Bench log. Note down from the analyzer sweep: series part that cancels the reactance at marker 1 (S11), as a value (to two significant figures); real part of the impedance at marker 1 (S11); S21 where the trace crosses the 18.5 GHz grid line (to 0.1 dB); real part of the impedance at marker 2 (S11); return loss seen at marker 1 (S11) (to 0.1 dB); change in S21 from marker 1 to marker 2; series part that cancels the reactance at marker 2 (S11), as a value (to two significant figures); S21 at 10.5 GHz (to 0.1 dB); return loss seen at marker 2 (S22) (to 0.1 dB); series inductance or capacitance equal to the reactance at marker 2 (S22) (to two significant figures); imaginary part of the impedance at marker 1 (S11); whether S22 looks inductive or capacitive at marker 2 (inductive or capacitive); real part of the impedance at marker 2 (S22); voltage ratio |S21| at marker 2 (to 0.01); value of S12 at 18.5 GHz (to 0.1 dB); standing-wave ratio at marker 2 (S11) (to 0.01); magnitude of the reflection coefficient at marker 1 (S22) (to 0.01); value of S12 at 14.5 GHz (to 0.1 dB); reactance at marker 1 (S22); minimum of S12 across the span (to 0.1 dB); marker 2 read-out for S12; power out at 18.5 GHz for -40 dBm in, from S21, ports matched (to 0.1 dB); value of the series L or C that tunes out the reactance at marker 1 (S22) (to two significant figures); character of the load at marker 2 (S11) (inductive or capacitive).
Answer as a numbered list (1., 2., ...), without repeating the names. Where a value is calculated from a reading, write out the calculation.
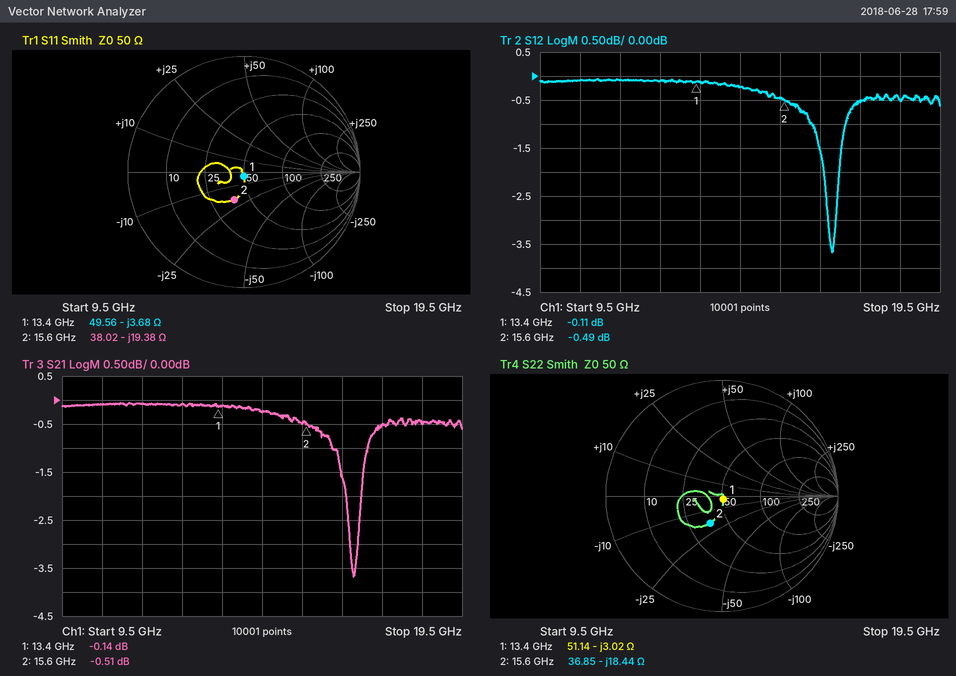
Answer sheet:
1. L = 3.68 Ω/(2π × 13.4 GHz) ≈ 44 pH
2. 49.56 Ω
3. -0.5 dB
4. 38.02 Ω
5. 28.6 dB
6. -0.51 − (-0.14) = -0.37 dB
7. L = 19.38 Ω/(2π × 15.6 GHz) ≈ 198 pH, so 200 pH to two significant figures
8. -0.1 dB
9. 11.9 dB
10. C = 1/(2π × 15.6 GHz × 18.44 Ω) ≈ 553 fF, so 550 fF to two significant figures
11. -3.68 Ω
12. capacitive
13. 36.85 Ω
14. 10^(-0.51/20) ≈ 0.94
15. -0.5 dB
16. 1.68
17. 0.03
18. -0.2 dB
19. -3.02 Ω
20. -3.7 dB
21. -0.49 dB
22. -40 dBm + (-0.5 dB) = -40.5 dBm
23. L = 3.02 Ω/(2π × 13.4 GHz) ≈ 36 pH
24. capacitive
